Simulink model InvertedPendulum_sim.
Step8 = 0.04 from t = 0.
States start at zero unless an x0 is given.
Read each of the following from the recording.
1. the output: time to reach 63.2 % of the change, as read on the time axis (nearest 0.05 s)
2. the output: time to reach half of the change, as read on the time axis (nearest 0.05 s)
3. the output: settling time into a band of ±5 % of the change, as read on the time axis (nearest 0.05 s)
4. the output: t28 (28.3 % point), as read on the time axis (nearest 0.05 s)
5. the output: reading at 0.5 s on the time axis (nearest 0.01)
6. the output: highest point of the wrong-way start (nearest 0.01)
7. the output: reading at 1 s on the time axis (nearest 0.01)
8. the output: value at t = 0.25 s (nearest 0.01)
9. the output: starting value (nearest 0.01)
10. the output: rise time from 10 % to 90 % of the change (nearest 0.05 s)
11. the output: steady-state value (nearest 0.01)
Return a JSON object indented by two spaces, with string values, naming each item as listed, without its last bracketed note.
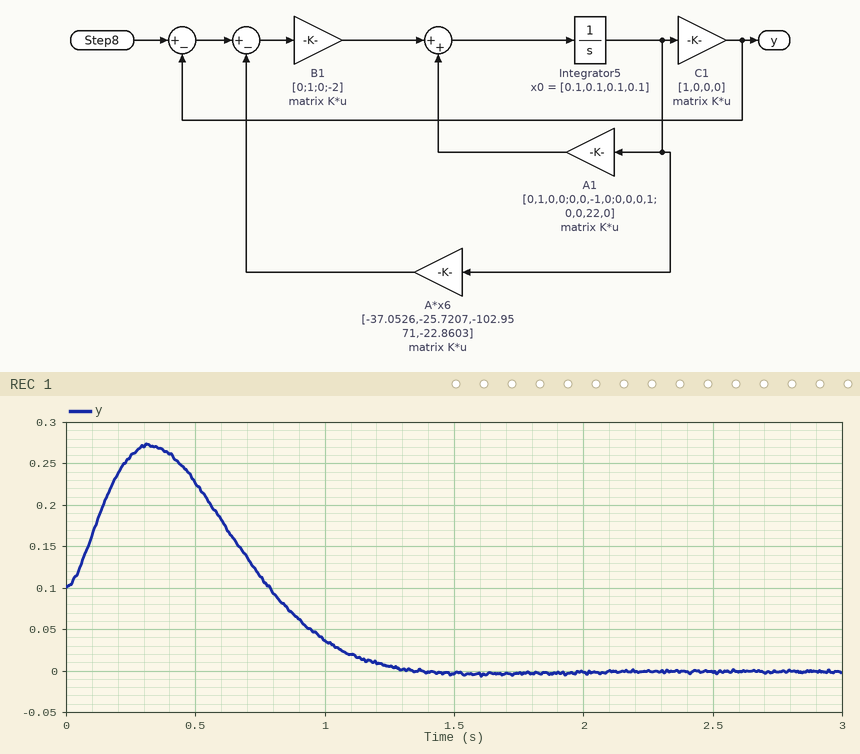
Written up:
{
  "the output: time to reach 63.2 % of the change, as read on the time axis": "1.00 s",
  "the output: time to reach half of the change, as read on the time axis": "0.95 s",
  "the output: settling time into a band of ±5 % of the change, as read on the time axis": "1.25 s",
  "the output: t28 (28.3 % point), as read on the time axis": "0.85 s",
  "the output: reading at 0.5 s on the time axis": "0.23",
  "the output: highest point of the wrong-way start": "0.27",
  "the output: reading at 1 s on the time axis": "0.04",
  "the output: value at t = 0.25 s": "0.26",
  "the output: starting value": "0.10",
  "the output: rise time from 10 % to 90 % of the change": "0.40 s",
  "the output: steady-state value": "0.00"
}
